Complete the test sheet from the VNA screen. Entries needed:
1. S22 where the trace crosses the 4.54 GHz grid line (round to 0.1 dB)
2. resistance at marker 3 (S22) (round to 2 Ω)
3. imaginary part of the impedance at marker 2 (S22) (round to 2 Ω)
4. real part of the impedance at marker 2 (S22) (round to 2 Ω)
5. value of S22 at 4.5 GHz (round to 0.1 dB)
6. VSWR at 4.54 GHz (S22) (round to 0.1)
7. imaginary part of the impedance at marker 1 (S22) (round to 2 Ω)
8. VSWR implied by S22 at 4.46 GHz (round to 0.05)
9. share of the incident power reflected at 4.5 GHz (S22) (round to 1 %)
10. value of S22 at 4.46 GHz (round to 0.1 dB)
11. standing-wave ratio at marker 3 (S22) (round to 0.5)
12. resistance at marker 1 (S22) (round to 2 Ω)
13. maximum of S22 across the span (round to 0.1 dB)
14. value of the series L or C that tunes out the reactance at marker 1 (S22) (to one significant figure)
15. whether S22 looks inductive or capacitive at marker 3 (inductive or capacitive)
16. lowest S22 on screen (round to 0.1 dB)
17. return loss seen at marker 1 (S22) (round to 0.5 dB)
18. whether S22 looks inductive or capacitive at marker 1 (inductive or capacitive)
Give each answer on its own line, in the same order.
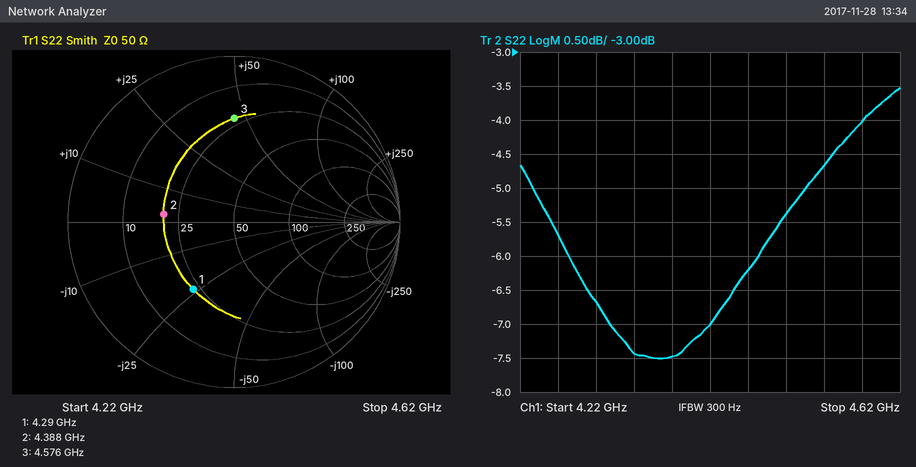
-4.7 dB
22 Ω
+2 Ω
20 Ω
-5.4 dB
3.8
-24 Ω
2.90
29 %
-6.2 dB
4.5
22 Ω
-3.5 dB
900 pH
inductive
-7.5 dB
6.5 dB
capacitive
